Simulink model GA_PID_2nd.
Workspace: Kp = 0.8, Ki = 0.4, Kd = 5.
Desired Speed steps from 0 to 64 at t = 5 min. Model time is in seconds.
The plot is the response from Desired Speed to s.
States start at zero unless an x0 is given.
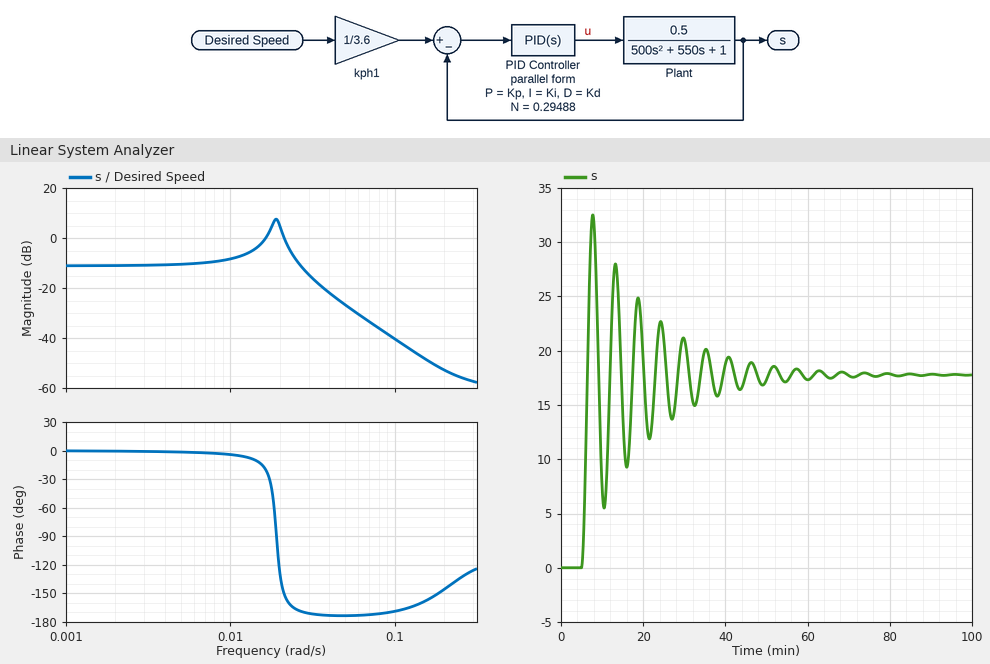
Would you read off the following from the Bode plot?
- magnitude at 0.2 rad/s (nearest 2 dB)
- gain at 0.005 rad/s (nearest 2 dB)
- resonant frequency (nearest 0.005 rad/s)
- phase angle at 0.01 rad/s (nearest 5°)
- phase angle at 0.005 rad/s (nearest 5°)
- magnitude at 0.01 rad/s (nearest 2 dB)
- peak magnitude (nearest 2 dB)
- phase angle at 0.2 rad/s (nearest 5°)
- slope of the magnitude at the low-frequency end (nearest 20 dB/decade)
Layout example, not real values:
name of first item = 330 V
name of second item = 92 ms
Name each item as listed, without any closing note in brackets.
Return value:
magnitude at 0.2 rad/s = -52 dB
gain at 0.005 rad/s = -10 dB
resonant frequency = 0.020 rad/s
phase angle at 0.01 rad/s = -5°
phase angle at 0.005 rad/s = 0°
magnitude at 0.01 rad/s = -8 dB
peak magnitude = 8 dB
phase angle at 0.2 rad/s = -145°
slope of the magnitude at the low-frequency end = 0 dB/decade
